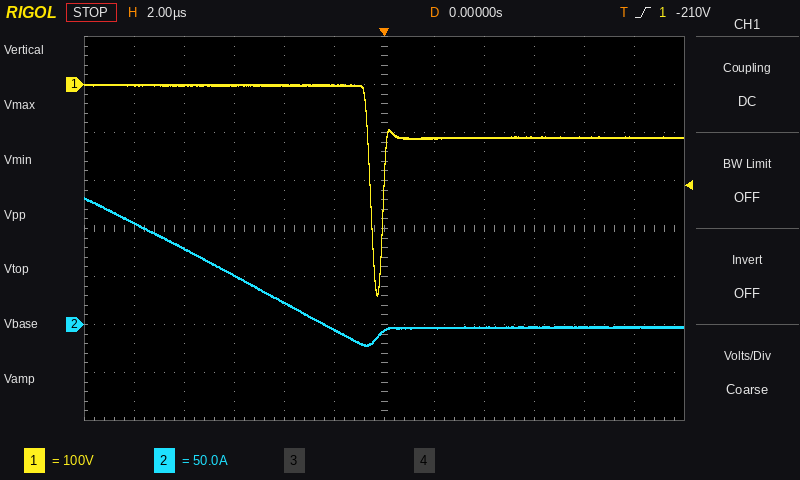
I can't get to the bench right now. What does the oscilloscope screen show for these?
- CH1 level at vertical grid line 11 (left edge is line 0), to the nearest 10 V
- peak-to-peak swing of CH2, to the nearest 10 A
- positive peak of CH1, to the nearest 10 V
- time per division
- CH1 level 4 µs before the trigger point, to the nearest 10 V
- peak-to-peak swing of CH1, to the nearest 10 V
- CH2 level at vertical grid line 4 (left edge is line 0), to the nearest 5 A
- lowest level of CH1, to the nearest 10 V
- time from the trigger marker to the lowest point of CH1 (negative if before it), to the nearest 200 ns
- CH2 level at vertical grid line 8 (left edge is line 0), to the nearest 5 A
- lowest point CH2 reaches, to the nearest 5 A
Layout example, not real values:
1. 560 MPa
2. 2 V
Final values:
1. -110 V
2. 150 A
3. 0 V
4. 2 µs
5. 0 V
6. 440 V
7. 25 A
8. -440 V
9. -200 ns
10. -5 A
11. -20 A
